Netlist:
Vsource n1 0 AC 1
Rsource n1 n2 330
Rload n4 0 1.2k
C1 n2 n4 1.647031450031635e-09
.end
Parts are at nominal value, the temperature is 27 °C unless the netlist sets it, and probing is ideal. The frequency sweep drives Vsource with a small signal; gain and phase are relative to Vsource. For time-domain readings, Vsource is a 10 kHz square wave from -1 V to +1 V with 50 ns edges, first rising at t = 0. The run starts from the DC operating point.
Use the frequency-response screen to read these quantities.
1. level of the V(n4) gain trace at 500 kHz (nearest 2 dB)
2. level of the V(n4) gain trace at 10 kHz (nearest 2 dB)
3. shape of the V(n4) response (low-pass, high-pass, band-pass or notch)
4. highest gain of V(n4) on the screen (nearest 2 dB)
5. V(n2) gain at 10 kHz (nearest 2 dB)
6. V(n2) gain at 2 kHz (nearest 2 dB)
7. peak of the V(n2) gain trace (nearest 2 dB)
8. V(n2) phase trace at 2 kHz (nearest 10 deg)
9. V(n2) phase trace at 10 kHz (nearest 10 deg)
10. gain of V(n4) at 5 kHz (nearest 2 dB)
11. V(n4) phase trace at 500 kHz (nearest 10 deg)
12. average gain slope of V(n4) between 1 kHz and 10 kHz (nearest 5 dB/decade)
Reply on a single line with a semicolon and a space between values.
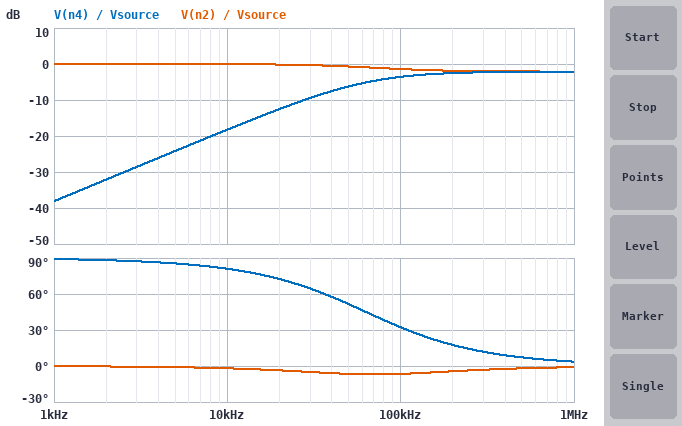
-2 dB; -18 dB; high-pass; -2 dB; 0 dB; 0 dB; 0 dB; 0 deg; 0 deg; -24 dB; 10 deg; 20 dB/decade
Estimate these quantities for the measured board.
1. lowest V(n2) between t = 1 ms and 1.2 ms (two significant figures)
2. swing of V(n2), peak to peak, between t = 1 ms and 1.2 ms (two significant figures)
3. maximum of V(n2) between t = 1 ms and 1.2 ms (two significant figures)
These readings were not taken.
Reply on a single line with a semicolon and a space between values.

-1.0 V; 2.0 V; 1.0 V
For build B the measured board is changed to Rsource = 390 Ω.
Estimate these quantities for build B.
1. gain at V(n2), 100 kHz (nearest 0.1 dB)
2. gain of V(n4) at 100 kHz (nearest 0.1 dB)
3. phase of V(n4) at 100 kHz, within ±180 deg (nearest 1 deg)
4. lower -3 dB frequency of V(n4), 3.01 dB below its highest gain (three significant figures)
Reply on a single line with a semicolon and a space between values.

-1.6 dB; -3.8 dB; 31 deg; 60.8 kHz
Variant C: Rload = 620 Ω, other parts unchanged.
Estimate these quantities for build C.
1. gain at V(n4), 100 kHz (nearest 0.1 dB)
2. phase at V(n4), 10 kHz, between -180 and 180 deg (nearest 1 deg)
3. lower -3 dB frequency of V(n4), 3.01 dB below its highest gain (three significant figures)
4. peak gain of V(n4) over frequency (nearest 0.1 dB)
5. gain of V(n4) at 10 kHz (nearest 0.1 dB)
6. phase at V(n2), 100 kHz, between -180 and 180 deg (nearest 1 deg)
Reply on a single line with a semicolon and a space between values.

-6.8 dB; 84 deg; 102 kHz; -3.7 dB; -23.9 dB; -12 deg
